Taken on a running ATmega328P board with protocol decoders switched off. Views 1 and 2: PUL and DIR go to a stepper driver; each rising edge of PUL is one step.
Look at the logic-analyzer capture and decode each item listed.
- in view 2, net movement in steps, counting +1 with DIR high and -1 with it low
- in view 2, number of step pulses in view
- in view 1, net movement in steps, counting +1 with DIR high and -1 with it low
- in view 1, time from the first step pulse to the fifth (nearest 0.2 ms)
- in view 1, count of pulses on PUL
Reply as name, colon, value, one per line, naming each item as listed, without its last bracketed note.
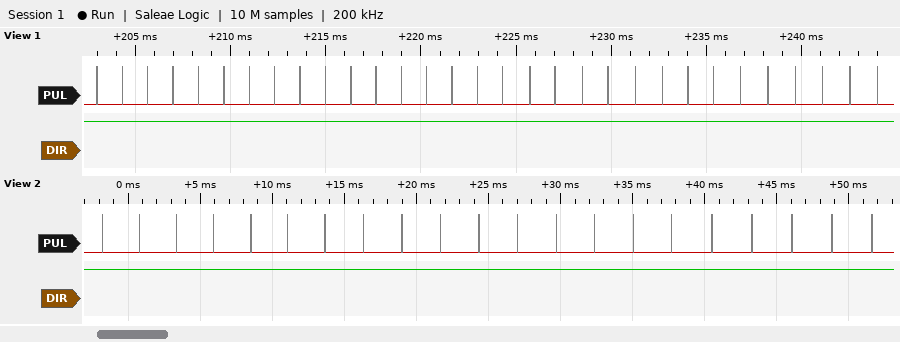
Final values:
in view 2, net movement in steps, counting +1 with DIR high and -1 with it low: +21
in view 2, number of step pulses in view: 21
in view 1, net movement in steps, counting +1 with DIR high and -1 with it low: +31
in view 1, time from the first step pulse to the fifth: 5.4 ms
in view 1, count of pulses on PUL: 31
